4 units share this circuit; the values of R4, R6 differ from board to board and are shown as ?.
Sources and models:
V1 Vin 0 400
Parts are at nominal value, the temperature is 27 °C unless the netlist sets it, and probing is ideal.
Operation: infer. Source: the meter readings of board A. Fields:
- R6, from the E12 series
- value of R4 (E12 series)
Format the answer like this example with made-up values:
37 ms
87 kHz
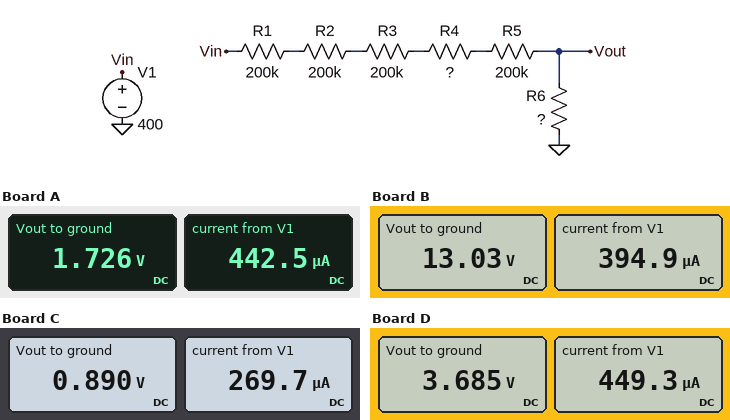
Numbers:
3.9 kΩ
100 kΩ
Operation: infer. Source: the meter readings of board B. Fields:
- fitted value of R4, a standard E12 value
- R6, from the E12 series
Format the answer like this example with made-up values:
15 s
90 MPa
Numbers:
180 kΩ
33 kΩ
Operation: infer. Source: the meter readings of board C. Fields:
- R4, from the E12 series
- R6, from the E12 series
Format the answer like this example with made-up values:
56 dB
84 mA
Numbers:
680 kΩ
3.3 kΩ
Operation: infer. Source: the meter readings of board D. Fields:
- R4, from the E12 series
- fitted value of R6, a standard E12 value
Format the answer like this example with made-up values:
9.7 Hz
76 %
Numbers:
82 kΩ
8.2 kΩ
